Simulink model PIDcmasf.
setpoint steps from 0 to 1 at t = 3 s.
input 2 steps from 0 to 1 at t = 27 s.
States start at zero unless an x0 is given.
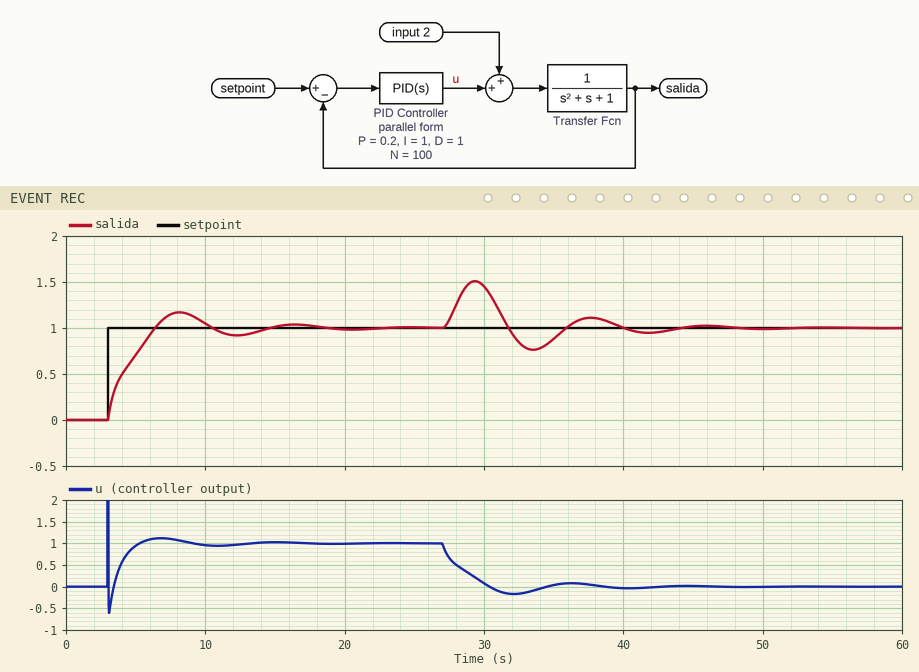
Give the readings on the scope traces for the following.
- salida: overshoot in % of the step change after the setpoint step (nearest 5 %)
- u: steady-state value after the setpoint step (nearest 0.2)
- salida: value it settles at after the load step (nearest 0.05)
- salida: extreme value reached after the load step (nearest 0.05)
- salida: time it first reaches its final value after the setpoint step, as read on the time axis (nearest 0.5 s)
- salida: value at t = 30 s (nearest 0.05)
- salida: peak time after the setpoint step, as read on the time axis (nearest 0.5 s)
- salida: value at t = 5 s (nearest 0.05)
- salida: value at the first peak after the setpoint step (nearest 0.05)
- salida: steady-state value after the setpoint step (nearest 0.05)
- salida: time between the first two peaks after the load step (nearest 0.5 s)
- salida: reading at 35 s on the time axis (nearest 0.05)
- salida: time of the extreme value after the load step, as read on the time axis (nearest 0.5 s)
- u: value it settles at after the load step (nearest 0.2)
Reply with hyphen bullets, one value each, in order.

- 15 %
- 1.0
- 1.00
- 1.50
- 6.5 s
- 1.45
- 8.0 s
- 0.70
- 1.15
- 1.00
- 8.5 s
- 0.90
- 29.5 s
- 0.0
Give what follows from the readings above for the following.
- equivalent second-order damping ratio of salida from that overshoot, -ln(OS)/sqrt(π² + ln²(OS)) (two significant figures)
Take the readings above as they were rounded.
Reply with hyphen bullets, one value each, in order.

- 0.52
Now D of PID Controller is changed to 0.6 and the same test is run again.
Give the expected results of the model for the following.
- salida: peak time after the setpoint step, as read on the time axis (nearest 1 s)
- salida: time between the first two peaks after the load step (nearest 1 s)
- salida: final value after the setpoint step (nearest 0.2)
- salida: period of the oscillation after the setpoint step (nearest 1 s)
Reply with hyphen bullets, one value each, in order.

- 7 s
- 7 s
- 1.0
- 7 s
